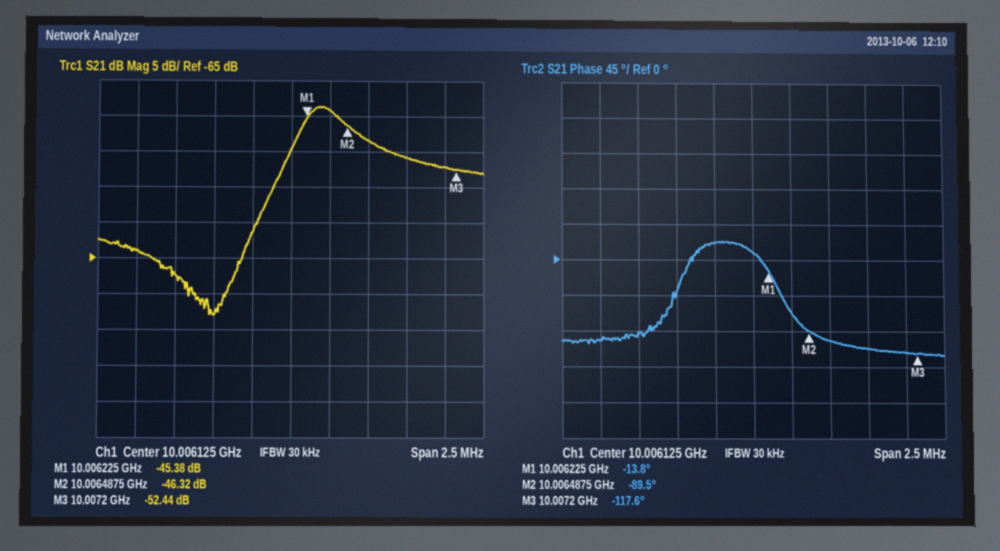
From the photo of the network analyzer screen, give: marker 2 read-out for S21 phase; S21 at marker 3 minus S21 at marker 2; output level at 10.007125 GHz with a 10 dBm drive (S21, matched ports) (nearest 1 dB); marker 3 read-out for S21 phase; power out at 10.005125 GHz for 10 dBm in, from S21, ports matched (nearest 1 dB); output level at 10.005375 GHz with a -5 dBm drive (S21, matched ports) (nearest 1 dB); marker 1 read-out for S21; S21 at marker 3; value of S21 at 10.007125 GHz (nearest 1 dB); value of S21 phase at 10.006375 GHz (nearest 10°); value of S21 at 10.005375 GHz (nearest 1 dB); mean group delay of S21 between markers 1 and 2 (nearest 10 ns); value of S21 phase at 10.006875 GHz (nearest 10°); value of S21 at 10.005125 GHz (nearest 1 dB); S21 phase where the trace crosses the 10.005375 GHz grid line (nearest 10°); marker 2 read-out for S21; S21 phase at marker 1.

-89.5°
-6.12 dB
-42 dBm
-117.6°
-54 dBm
-72 dBm
-45.38 dB
-52.44 dB
-52 dB
-70°
-67 dB
800 ns
-110°
-64 dB
-90°
-46.32 dB
-13.8°
